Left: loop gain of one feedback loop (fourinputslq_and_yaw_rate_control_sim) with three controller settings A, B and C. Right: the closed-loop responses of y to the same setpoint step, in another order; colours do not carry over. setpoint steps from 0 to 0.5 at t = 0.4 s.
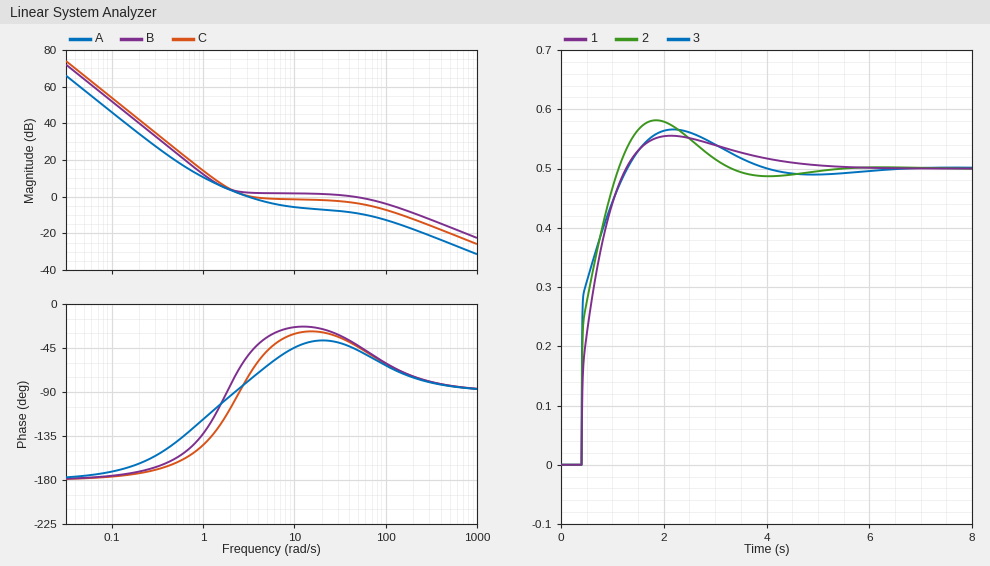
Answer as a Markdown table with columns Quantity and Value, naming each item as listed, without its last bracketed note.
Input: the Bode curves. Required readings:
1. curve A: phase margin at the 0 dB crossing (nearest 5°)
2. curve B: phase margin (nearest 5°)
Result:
| Quantity | Value |
|---|---|
| curve A: phase margin at the 0 dB crossing | 100° |
| curve B: phase margin | 140° |
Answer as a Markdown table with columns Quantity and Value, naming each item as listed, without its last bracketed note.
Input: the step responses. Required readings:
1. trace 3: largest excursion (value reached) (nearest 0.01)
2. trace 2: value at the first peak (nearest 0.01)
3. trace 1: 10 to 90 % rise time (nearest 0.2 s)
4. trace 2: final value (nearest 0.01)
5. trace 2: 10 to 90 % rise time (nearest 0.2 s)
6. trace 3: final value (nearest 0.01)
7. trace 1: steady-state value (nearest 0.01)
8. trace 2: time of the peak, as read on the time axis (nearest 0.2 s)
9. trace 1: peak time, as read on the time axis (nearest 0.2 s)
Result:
| Quantity | Value |
|---|---|
| trace 3: largest excursion (value reached) | 0.57 |
| trace 2: value at the first peak | 0.58 |
| trace 1: 10 to 90 % rise time | 0.6 s |
| trace 2: final value | 0.50 |
| trace 2: 10 to 90 % rise time | 0.6 s |
| trace 3: final value | 0.50 |
| trace 1: steady-state value | 0.50 |
| trace 2: time of the peak, as read on the time axis | 1.8 s |
| trace 1: peak time, as read on the time axis | 2.2 s |
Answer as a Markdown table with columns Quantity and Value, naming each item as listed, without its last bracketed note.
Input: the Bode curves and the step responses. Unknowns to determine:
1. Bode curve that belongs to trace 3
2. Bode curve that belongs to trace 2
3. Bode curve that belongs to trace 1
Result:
| Quantity | Value |
|---|---|
| Bode curve that belongs to trace 3 | B |
| Bode curve that belongs to trace 2 | C |
| Bode curve that belongs to trace 1 | A |
